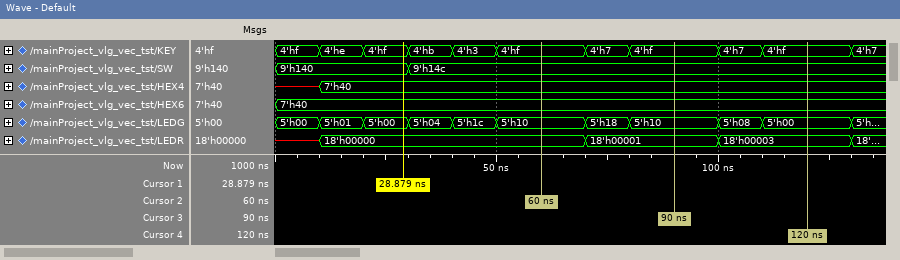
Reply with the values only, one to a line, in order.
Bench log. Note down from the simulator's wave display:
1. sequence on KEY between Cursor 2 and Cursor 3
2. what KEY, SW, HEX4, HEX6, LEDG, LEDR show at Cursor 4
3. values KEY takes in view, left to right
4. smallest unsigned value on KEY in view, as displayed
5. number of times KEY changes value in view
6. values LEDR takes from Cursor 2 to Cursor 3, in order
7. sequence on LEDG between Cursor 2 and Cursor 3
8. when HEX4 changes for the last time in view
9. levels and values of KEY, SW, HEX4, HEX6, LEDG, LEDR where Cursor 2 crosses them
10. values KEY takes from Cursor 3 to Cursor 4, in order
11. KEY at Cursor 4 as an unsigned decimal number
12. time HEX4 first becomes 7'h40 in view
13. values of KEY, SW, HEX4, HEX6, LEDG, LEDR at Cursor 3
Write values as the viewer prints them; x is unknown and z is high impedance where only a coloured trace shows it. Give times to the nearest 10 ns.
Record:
4'hf, 4'h7, 4'hf
KEY=4'hf, SW=9'h14c, HEX4=7'h40, HEX6=7'h40, LEDG=5'h00, LEDR=18'h00003
4'hf, 4'he, 4'hf, 4'hb, 4'h3, 4'hf, 4'h7, 4'hf, 4'h7, 4'hf, 4'h7
4'h3
10
18'h00000, 18'h00001
5'h10, 5'h18, 5'h10
10 ns
KEY=4'hf, SW=9'h14c, HEX4=7'h40, HEX6=7'h40, LEDG=5'h10, LEDR=18'h00000
4'hf, 4'h7, 4'hf
15
10 ns
KEY=4'hf, SW=9'h14c, HEX4=7'h40, HEX6=7'h40, LEDG=5'h10, LEDR=18'h00001
